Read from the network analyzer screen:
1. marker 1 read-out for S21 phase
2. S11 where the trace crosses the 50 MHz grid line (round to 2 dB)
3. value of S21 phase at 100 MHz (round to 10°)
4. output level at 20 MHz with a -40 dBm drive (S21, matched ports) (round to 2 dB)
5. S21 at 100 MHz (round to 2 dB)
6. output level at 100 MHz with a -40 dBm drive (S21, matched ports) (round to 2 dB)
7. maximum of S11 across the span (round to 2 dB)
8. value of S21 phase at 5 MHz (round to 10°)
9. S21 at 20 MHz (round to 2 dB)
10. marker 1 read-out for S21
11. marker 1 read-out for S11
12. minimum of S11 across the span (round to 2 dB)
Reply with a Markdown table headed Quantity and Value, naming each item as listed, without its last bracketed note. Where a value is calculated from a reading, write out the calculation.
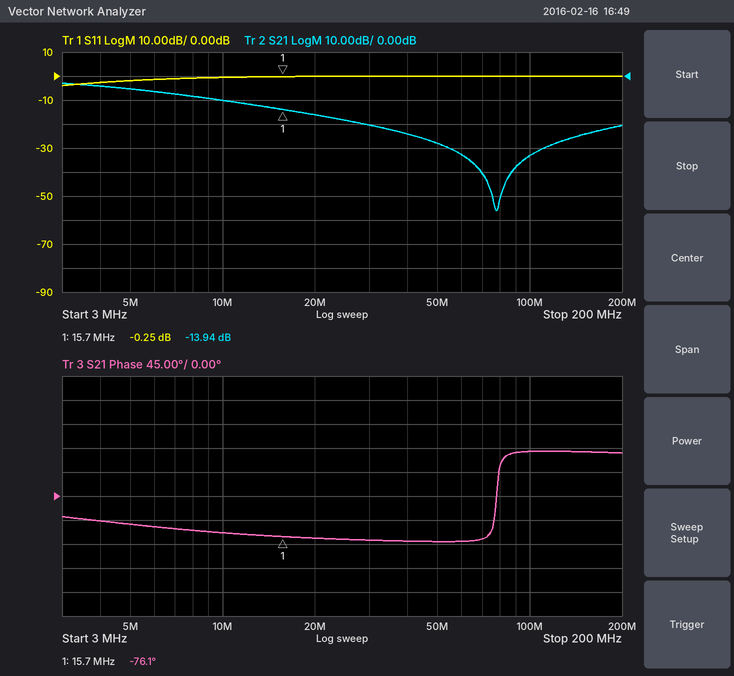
| Quantity | Value |
|---|---|
| marker 1 read-out for S21 phase | -76.1° |
| S11 where the trace crosses the 50 MHz grid line | 0 dB |
| value of S21 phase at 100 MHz | 80° |
| output level at 20 MHz with a -40 dBm drive (S21, matched ports) | -40 dBm + (-16 dB) = -56 dBm |
| S21 at 100 MHz | -34 dB |
| output level at 100 MHz with a -40 dBm drive (S21, matched ports) | -40 dBm + (-34 dB) = -74 dBm |
| maximum of S11 across the span | 0 dB |
| value of S21 phase at 5 MHz | -50° |
| S21 at 20 MHz | -16 dB |
| marker 1 read-out for S21 | -13.94 dB |
| marker 1 read-out for S11 | -0.25 dB |
| minimum of S11 across the span | -4 dB |
